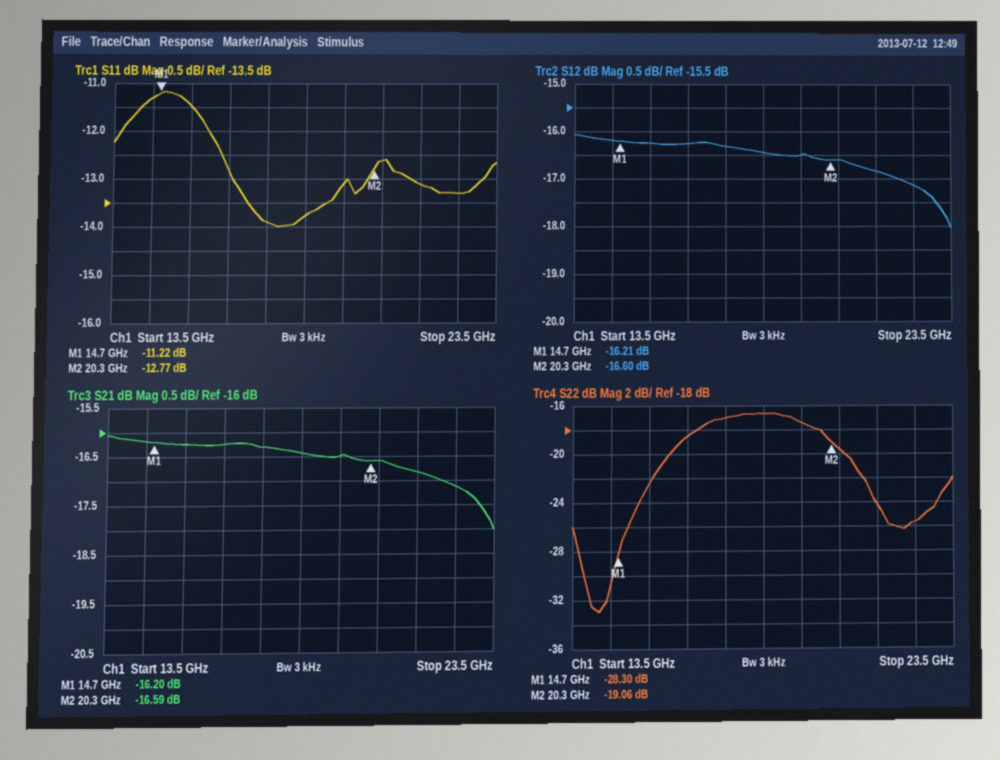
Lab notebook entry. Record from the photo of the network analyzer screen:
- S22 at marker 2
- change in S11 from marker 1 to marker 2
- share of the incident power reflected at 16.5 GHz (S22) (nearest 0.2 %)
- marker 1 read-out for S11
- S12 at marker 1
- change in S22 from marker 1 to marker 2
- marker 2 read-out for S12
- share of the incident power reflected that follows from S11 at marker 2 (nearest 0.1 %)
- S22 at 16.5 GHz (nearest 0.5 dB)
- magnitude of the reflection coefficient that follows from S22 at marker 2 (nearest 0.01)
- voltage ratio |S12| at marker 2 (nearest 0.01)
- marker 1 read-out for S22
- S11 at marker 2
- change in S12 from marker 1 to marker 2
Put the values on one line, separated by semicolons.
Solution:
-19.06 dB; -1.55 dB; 1.4 %; -11.22 dB; -16.21 dB; 9.24 dB; -16.60 dB; 5.3 %; -18.5 dB; 0.11; 0.15; -28.30 dB; -12.77 dB; -0.39 dB
